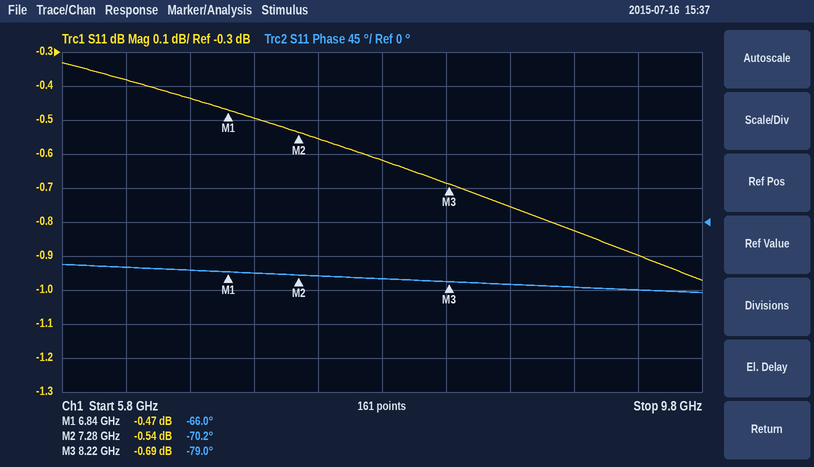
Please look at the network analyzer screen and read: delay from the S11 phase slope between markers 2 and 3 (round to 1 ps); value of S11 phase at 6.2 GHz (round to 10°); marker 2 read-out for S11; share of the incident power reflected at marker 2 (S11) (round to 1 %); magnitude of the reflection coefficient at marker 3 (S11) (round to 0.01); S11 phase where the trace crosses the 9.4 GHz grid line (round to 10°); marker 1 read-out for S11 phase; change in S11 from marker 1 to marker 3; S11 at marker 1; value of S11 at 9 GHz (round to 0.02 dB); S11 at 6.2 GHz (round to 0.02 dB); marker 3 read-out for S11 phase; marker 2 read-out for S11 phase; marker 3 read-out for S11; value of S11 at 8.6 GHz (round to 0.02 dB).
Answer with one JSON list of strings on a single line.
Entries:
["26 ps", "-60°", "-0.54 dB", "88 %", "0.92", "-90°", "-66.0°", "-0.22 dB", "-0.47 dB", "-0.82 dB", "-0.38 dB", "-79.0°", "-70.2°", "-0.69 dB", "-0.76 dB"]
